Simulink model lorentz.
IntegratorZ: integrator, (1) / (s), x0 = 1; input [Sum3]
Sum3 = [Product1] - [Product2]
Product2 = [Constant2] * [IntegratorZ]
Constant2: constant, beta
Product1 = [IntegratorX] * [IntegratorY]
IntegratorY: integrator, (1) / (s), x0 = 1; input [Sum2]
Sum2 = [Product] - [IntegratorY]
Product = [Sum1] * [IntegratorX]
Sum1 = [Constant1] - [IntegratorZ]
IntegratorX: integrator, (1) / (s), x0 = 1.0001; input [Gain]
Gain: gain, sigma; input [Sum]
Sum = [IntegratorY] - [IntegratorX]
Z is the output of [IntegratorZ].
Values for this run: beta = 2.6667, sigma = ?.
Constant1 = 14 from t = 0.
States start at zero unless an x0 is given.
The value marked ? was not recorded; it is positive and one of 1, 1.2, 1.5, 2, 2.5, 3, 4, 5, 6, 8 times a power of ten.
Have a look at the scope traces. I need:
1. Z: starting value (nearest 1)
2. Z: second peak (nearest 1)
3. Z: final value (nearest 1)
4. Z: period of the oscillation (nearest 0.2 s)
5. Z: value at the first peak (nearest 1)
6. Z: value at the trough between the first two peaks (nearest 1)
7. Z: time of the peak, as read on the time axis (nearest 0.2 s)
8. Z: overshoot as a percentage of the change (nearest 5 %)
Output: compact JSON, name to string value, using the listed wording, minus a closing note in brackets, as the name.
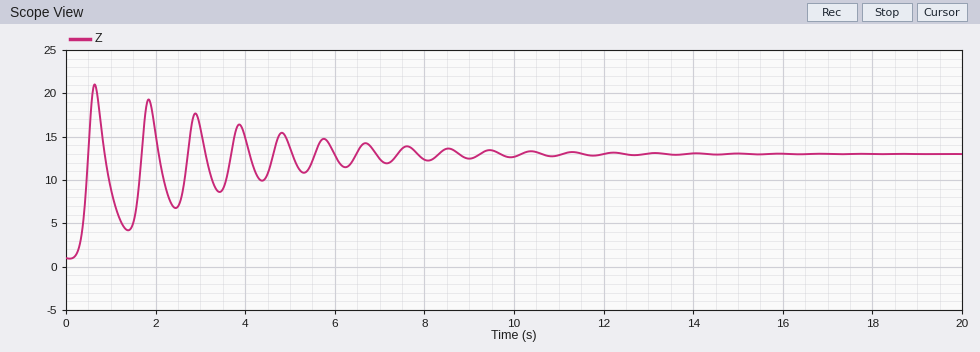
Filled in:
{"Z: starting value": "1", "Z: second peak": "19", "Z: final value": "13", "Z: period of the oscillation": "1.2 s", "Z: value at the first peak": "21", "Z: value at the trough between the first two peaks": "4", "Z: time of the peak, as read on the time axis": "0.6 s", "Z: overshoot as a percentage of the change": "65 %"}
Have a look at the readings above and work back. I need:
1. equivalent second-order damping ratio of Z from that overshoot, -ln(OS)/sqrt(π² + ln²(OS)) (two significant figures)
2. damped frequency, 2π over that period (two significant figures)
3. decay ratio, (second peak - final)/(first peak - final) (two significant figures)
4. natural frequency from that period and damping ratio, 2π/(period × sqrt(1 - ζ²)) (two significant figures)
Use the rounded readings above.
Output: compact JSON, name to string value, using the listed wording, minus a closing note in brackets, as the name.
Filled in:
{"equivalent second-order damping ratio of Z from that overshoot, -ln(OS)/sqrt(π² + ln²(OS))": "0.14", "damped frequency, 2π over that period": "5.2 rad/s", "decay ratio, (second peak - final)/(first peak - final)": "0.75", "natural frequency from that period and damping ratio, 2π/(period × sqrt(1 - ζ²))": "5.3 rad/s"}
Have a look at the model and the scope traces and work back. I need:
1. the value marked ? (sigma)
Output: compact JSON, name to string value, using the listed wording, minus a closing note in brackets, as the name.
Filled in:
{"the value marked ?": "6"}
